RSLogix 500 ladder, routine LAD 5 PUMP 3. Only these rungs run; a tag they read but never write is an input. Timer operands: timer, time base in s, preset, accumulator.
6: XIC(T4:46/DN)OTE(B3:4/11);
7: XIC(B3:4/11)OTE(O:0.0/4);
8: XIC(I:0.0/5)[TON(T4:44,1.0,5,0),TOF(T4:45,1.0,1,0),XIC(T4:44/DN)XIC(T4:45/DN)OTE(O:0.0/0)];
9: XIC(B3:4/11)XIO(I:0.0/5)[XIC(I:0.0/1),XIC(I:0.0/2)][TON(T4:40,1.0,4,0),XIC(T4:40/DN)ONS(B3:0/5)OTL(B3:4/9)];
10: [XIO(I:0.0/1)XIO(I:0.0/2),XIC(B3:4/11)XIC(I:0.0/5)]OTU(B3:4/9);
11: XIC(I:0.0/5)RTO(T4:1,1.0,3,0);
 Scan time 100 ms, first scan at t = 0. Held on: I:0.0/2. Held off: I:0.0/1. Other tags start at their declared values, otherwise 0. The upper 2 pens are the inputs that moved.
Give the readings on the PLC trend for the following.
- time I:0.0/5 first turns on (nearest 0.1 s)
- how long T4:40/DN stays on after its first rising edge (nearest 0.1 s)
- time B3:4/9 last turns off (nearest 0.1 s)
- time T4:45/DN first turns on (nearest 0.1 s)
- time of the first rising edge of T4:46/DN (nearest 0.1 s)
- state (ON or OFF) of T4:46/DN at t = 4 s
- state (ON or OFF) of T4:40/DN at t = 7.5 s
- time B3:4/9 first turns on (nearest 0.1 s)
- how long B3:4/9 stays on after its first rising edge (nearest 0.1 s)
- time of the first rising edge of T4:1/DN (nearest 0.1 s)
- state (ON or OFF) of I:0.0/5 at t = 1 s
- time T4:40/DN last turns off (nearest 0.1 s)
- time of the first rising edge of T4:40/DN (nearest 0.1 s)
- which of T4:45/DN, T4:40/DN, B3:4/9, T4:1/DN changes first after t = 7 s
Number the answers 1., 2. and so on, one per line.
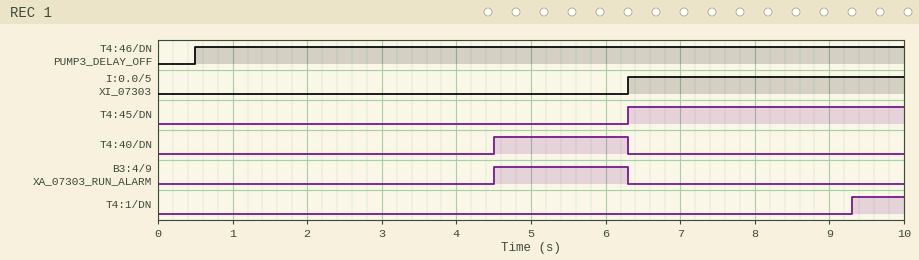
1. 6.3 s
2. 1.8 s
3. 6.3 s
4. 6.3 s
5. 0.5 s
6. ON
7. OFF
8. 4.5 s
9. 1.8 s
10. 9.3 s
11. OFF
12. 6.3 s
13. 4.5 s
14. T4:1/DN
